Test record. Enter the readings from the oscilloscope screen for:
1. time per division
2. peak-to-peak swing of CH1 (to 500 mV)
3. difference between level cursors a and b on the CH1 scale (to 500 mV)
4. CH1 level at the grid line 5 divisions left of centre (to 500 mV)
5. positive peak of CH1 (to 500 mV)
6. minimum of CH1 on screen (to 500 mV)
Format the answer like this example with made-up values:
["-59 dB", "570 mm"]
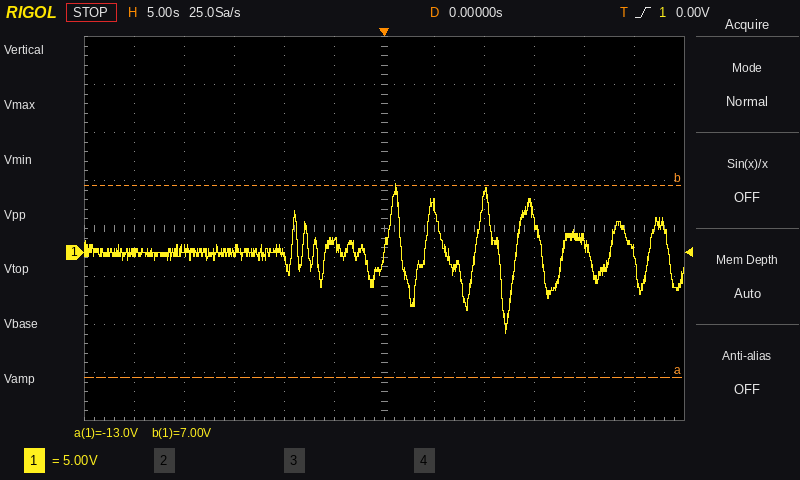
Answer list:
["5 s", "15.5 V", "20.0 V", "0.0 V", "7.0 V", "-8.5 V"]
